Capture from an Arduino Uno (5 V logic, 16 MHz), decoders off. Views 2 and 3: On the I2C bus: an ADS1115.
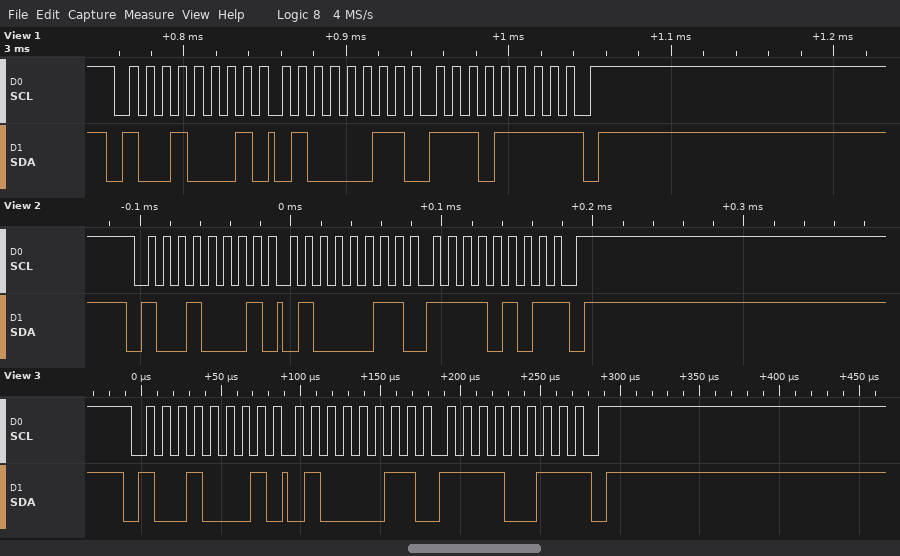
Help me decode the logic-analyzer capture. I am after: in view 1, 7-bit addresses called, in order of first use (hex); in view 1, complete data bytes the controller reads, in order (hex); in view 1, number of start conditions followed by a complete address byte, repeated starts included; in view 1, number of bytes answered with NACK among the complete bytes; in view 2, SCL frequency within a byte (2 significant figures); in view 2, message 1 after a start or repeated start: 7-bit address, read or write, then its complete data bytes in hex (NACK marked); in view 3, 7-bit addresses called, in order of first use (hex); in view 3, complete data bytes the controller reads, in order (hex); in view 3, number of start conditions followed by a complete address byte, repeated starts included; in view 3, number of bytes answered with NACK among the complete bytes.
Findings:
0x48
43 EF
1
1
100 kHz
0x48 read: 43 F5 NACK
0x48
43 F3
1
1
